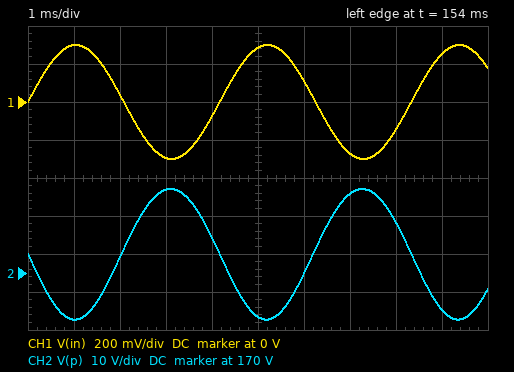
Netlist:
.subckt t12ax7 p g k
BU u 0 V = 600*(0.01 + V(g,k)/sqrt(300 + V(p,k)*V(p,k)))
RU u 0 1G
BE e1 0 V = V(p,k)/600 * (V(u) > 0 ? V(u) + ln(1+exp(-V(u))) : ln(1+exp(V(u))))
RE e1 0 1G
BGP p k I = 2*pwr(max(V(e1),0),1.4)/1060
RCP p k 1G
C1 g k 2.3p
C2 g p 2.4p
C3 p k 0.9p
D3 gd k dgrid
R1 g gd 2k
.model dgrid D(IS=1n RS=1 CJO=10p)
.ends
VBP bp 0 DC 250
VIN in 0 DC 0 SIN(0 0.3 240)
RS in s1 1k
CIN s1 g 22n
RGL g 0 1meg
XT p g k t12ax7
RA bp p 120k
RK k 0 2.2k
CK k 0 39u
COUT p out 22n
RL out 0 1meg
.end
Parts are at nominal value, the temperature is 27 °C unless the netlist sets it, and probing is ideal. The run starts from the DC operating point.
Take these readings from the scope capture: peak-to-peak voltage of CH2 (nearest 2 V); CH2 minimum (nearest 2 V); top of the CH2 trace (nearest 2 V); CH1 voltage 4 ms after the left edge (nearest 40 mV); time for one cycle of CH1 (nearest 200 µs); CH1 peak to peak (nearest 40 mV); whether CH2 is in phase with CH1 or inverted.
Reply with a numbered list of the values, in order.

1. 34 V
2. 158 V
3. 192 V
4. -80 mV
5. 4.2 ms
6. 600 mV
7. inverted
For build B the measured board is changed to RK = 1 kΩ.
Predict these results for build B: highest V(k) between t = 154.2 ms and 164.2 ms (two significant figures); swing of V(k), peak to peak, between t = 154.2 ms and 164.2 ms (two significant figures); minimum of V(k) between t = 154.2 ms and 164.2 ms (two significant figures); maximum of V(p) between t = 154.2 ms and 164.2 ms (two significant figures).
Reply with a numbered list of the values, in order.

1. 890 mV
2. 6.1 mV
3. 880 mV
4. 160 V
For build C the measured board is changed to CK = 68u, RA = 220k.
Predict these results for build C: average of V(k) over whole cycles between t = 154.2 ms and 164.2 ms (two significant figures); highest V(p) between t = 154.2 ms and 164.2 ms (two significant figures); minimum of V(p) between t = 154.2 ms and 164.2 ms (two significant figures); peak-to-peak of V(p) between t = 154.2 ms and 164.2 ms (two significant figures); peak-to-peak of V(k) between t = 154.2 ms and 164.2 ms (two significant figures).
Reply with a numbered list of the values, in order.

1. 1.1 V
2. 160 V
3. 120 V
4. 40 V
5. 2.2 mV
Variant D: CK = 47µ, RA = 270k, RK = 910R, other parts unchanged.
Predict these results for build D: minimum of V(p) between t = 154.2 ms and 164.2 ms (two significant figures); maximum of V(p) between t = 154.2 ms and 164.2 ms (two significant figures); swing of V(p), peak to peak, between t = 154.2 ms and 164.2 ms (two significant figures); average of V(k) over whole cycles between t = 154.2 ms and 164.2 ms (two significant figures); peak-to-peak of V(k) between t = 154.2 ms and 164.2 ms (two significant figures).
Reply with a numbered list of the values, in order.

1. 71 V
2. 120 V
3. 45 V
4. 530 mV
5. 3.0 mV
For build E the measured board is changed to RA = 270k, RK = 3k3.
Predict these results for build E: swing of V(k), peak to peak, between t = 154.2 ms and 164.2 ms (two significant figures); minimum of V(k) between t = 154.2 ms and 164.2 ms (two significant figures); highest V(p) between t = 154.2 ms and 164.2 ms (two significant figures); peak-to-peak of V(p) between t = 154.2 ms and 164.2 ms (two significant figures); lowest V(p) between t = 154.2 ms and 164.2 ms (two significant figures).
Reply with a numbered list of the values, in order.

1. 3.1 mV
2. 1.2 V
3. 170 V
4. 39 V
5. 130 V
